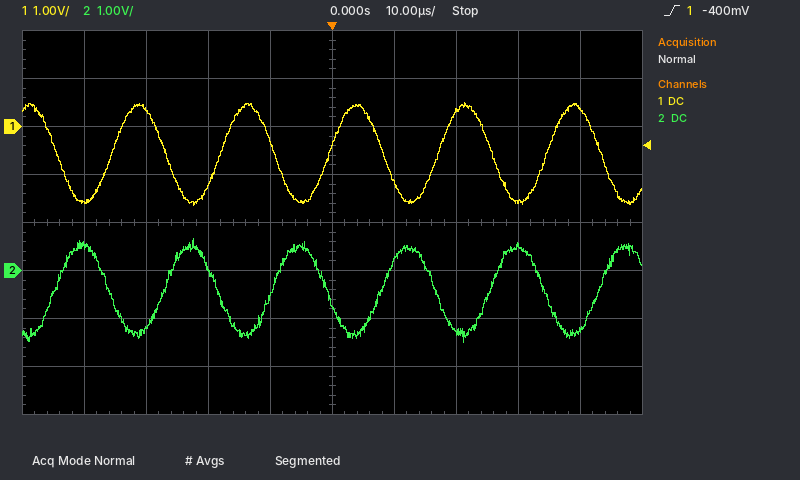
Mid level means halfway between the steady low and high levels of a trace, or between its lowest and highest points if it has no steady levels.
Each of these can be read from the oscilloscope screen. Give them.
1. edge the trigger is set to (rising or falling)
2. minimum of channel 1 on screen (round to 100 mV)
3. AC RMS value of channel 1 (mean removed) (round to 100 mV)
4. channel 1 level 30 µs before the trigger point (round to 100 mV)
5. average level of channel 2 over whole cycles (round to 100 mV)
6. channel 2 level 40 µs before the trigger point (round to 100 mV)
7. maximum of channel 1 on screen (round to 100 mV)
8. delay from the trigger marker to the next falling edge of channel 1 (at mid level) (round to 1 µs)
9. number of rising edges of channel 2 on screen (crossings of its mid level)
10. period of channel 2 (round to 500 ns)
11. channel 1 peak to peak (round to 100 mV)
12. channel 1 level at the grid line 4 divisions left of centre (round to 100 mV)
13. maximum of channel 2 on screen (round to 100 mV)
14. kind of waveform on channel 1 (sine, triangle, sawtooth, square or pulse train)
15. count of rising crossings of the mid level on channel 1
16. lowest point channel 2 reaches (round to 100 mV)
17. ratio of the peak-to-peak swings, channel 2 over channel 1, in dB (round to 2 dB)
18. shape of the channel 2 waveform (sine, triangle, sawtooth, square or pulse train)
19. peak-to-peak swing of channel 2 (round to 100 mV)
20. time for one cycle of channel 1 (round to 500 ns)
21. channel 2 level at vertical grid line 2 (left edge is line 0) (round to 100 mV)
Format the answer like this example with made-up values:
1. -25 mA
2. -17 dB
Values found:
1. rising
2. -1.6 V
3. 700 mV
4. 400 mV
5. -400 mV
6. 500 mV
7. 500 mV
8. 8 µs
9. 6
10. 17.5 µs
11. 2.1 V
12. -1.6 V
13. 700 mV
14. sine
15. 5
16. -1.5 V
17. 0 dB
18. sine
19. 2.2 V
20. 17.5 µs
21. -1.2 V
